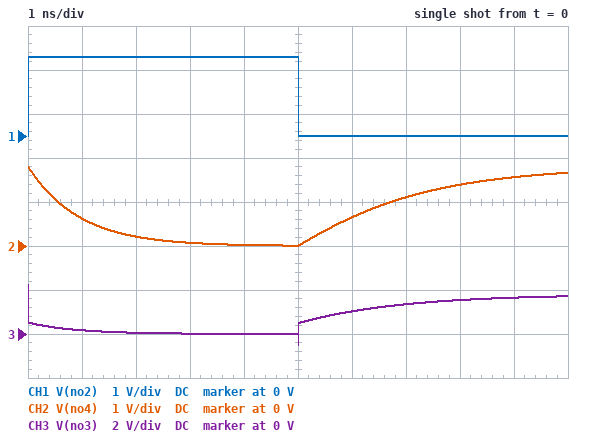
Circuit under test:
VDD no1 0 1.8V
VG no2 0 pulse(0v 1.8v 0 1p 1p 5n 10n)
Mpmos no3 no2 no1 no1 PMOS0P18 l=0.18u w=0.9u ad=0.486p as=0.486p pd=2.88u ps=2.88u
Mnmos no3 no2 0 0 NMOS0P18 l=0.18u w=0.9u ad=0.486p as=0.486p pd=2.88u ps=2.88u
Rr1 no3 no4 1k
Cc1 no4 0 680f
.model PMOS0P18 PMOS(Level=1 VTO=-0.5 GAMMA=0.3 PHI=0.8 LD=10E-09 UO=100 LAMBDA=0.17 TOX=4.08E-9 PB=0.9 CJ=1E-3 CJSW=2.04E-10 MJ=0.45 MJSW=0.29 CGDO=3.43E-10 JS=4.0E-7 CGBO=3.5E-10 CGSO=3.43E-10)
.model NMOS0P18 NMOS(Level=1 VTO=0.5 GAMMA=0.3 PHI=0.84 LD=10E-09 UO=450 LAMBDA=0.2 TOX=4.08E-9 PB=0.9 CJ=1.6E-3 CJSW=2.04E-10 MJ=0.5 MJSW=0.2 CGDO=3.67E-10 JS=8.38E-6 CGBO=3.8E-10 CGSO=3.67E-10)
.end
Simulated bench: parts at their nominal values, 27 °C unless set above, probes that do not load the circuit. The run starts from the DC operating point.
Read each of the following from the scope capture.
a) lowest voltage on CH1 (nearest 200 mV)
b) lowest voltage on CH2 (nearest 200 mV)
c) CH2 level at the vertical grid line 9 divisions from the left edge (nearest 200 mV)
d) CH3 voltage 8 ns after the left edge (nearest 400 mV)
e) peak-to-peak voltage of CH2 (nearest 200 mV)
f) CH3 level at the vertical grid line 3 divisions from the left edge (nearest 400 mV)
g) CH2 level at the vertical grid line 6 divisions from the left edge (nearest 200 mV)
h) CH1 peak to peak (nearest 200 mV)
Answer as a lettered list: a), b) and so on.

a) 0 V
b) 0 V
c) 1.6 V
d) 1.6 V
e) 1.8 V
f) 0 V
g) 600 mV
h) 1.8 V
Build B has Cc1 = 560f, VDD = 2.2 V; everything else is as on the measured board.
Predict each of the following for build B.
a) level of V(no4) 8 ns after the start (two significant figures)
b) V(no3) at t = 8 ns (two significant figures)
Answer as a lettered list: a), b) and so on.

a) 2.0 V
b) 2.1 V
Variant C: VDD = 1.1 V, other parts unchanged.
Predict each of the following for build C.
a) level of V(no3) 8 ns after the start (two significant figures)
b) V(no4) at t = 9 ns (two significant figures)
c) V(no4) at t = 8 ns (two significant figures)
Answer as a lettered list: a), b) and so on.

a) 520 mV
b) 560 mV
c) 430 mV
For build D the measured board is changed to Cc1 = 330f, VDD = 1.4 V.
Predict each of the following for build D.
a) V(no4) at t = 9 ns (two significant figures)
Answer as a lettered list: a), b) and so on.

a) 1.3 V
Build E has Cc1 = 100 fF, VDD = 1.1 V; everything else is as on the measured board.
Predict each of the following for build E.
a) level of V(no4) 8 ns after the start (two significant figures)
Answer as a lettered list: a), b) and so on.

a) 1.1 V
